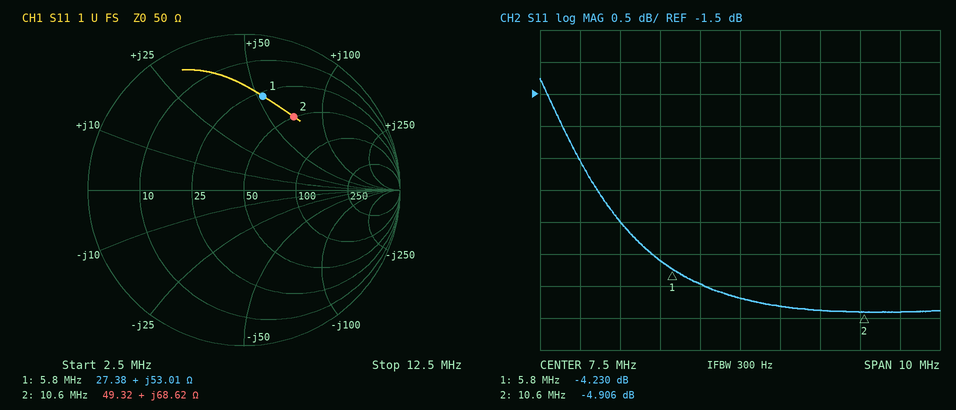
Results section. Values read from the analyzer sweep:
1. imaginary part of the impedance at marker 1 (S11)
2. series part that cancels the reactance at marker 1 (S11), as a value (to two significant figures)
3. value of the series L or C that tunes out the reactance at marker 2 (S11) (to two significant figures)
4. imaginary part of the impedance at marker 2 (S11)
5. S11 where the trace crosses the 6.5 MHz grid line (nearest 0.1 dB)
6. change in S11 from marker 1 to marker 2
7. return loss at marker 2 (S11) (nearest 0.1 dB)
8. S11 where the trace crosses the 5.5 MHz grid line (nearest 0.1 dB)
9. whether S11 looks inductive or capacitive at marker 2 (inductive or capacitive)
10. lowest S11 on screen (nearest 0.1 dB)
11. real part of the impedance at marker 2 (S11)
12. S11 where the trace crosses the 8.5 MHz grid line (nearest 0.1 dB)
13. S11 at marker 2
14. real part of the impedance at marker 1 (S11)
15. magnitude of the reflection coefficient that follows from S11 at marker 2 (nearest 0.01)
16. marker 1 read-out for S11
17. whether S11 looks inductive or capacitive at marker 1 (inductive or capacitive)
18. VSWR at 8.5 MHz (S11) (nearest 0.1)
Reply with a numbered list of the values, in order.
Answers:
1. +53.01 Ω
2. 520 pF
3. 220 pF
4. +68.62 Ω
5. -4.5 dB
6. -0.676 dB
7. 4.9 dB
8. -4.1 dB
9. inductive
10. -4.9 dB
11. 49.32 Ω
12. -4.8 dB
13. -4.906 dB
14. 27.38 Ω
15. 0.57
16. -4.230 dB
17. inductive
18. 3.7
